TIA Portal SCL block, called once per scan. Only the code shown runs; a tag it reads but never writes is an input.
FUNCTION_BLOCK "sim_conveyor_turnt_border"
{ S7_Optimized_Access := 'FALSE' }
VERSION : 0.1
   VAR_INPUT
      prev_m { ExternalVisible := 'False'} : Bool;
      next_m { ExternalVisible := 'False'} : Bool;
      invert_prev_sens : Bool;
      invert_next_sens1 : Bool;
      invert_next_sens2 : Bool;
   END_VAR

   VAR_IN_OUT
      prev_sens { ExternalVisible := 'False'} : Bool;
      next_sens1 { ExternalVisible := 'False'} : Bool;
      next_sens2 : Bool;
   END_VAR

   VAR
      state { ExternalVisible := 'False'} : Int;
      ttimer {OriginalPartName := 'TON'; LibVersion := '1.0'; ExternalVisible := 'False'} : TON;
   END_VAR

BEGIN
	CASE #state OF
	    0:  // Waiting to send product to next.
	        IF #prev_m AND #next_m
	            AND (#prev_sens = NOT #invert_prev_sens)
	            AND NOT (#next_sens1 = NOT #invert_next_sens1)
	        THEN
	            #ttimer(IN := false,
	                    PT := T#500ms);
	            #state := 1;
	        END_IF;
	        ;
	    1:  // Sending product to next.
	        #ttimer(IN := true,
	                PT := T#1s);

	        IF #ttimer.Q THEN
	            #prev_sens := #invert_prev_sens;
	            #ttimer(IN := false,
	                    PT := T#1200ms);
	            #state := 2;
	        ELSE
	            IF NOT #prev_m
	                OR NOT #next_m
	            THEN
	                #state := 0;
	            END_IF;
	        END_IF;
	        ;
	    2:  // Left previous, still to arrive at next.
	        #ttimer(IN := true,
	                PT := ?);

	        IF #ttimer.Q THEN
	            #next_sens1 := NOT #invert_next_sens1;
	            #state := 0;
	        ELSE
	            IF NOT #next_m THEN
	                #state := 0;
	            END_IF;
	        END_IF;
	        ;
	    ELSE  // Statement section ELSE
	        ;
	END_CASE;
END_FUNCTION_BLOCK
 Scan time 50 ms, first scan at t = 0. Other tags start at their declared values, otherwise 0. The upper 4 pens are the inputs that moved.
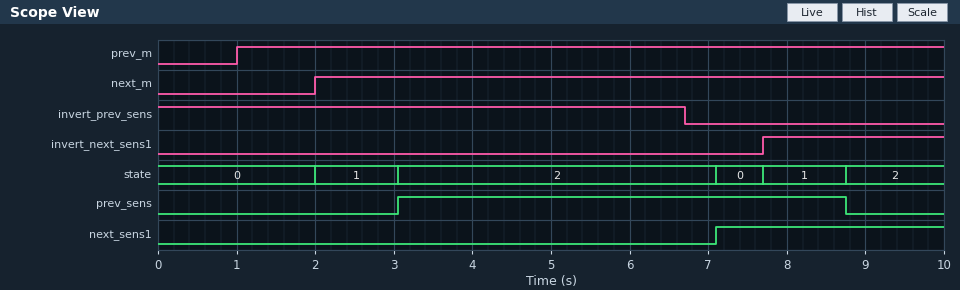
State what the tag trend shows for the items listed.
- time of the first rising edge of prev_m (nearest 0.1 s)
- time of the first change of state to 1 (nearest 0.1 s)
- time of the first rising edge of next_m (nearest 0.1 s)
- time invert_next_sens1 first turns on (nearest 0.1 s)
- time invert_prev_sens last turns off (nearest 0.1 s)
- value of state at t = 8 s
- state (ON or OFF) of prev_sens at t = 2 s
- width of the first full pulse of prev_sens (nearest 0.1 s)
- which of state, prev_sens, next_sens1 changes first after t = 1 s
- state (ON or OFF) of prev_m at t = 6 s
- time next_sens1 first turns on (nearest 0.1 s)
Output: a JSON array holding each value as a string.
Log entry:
["1.0 s", "2.0 s", "2.0 s", "7.7 s", "6.7 s", "1", "OFF", "5.7 s", "state", "ON", "7.1 s"]
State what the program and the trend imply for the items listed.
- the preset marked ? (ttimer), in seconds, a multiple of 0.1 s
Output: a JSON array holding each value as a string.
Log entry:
["4.0 s"]
